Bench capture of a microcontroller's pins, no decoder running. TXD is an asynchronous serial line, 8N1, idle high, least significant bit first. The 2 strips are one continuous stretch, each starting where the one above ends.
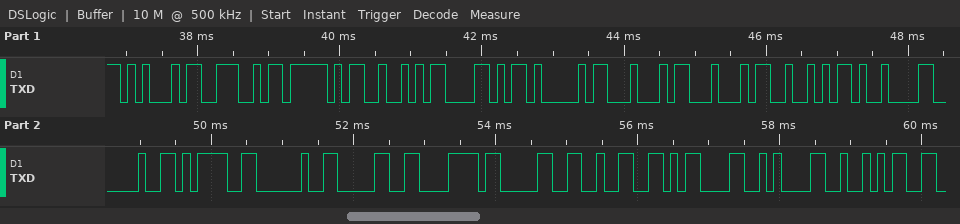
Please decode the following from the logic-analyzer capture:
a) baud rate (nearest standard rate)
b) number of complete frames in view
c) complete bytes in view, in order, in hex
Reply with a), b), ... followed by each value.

a) 9600 baud
b) 20
c) 45 4E 5F 52 58 41 44 44 52 09 20 3D 20 30 78 30 32 0D 0A 52
